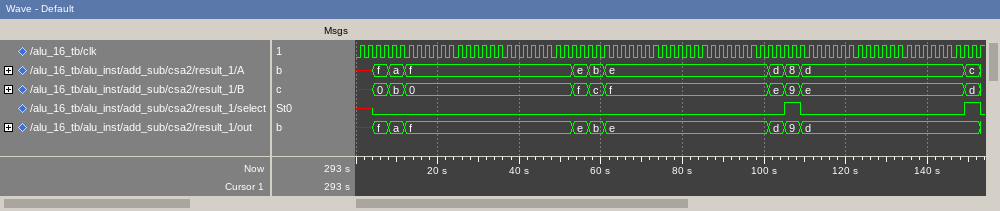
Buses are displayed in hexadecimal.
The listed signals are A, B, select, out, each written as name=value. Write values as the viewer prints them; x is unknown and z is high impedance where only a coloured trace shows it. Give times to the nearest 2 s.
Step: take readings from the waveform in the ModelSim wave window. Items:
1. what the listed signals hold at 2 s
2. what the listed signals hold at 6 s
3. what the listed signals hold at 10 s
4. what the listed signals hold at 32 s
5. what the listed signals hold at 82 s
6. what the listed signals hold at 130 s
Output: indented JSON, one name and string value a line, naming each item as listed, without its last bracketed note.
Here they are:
{
  "what the listed signals hold at 2 s": "A=x, B=x, select=x, out=x",
  "what the listed signals hold at 6 s": "A=f, B=0, select=0, out=f",
  "what the listed signals hold at 10 s": "A=a, B=b, select=0, out=a",
  "what the listed signals hold at 32 s": "A=f, B=0, select=0, out=f",
  "what the listed signals hold at 82 s": "A=e, B=f, select=0, out=e",
  "what the listed signals hold at 130 s": "A=d, B=e, select=0, out=d"
}
